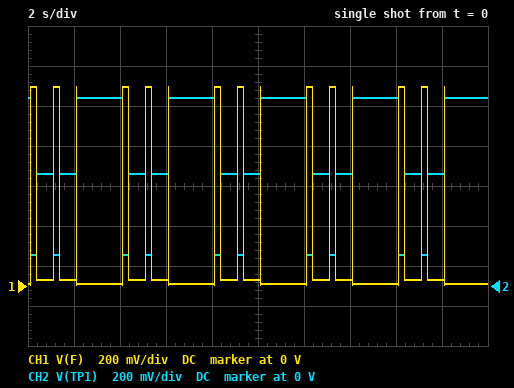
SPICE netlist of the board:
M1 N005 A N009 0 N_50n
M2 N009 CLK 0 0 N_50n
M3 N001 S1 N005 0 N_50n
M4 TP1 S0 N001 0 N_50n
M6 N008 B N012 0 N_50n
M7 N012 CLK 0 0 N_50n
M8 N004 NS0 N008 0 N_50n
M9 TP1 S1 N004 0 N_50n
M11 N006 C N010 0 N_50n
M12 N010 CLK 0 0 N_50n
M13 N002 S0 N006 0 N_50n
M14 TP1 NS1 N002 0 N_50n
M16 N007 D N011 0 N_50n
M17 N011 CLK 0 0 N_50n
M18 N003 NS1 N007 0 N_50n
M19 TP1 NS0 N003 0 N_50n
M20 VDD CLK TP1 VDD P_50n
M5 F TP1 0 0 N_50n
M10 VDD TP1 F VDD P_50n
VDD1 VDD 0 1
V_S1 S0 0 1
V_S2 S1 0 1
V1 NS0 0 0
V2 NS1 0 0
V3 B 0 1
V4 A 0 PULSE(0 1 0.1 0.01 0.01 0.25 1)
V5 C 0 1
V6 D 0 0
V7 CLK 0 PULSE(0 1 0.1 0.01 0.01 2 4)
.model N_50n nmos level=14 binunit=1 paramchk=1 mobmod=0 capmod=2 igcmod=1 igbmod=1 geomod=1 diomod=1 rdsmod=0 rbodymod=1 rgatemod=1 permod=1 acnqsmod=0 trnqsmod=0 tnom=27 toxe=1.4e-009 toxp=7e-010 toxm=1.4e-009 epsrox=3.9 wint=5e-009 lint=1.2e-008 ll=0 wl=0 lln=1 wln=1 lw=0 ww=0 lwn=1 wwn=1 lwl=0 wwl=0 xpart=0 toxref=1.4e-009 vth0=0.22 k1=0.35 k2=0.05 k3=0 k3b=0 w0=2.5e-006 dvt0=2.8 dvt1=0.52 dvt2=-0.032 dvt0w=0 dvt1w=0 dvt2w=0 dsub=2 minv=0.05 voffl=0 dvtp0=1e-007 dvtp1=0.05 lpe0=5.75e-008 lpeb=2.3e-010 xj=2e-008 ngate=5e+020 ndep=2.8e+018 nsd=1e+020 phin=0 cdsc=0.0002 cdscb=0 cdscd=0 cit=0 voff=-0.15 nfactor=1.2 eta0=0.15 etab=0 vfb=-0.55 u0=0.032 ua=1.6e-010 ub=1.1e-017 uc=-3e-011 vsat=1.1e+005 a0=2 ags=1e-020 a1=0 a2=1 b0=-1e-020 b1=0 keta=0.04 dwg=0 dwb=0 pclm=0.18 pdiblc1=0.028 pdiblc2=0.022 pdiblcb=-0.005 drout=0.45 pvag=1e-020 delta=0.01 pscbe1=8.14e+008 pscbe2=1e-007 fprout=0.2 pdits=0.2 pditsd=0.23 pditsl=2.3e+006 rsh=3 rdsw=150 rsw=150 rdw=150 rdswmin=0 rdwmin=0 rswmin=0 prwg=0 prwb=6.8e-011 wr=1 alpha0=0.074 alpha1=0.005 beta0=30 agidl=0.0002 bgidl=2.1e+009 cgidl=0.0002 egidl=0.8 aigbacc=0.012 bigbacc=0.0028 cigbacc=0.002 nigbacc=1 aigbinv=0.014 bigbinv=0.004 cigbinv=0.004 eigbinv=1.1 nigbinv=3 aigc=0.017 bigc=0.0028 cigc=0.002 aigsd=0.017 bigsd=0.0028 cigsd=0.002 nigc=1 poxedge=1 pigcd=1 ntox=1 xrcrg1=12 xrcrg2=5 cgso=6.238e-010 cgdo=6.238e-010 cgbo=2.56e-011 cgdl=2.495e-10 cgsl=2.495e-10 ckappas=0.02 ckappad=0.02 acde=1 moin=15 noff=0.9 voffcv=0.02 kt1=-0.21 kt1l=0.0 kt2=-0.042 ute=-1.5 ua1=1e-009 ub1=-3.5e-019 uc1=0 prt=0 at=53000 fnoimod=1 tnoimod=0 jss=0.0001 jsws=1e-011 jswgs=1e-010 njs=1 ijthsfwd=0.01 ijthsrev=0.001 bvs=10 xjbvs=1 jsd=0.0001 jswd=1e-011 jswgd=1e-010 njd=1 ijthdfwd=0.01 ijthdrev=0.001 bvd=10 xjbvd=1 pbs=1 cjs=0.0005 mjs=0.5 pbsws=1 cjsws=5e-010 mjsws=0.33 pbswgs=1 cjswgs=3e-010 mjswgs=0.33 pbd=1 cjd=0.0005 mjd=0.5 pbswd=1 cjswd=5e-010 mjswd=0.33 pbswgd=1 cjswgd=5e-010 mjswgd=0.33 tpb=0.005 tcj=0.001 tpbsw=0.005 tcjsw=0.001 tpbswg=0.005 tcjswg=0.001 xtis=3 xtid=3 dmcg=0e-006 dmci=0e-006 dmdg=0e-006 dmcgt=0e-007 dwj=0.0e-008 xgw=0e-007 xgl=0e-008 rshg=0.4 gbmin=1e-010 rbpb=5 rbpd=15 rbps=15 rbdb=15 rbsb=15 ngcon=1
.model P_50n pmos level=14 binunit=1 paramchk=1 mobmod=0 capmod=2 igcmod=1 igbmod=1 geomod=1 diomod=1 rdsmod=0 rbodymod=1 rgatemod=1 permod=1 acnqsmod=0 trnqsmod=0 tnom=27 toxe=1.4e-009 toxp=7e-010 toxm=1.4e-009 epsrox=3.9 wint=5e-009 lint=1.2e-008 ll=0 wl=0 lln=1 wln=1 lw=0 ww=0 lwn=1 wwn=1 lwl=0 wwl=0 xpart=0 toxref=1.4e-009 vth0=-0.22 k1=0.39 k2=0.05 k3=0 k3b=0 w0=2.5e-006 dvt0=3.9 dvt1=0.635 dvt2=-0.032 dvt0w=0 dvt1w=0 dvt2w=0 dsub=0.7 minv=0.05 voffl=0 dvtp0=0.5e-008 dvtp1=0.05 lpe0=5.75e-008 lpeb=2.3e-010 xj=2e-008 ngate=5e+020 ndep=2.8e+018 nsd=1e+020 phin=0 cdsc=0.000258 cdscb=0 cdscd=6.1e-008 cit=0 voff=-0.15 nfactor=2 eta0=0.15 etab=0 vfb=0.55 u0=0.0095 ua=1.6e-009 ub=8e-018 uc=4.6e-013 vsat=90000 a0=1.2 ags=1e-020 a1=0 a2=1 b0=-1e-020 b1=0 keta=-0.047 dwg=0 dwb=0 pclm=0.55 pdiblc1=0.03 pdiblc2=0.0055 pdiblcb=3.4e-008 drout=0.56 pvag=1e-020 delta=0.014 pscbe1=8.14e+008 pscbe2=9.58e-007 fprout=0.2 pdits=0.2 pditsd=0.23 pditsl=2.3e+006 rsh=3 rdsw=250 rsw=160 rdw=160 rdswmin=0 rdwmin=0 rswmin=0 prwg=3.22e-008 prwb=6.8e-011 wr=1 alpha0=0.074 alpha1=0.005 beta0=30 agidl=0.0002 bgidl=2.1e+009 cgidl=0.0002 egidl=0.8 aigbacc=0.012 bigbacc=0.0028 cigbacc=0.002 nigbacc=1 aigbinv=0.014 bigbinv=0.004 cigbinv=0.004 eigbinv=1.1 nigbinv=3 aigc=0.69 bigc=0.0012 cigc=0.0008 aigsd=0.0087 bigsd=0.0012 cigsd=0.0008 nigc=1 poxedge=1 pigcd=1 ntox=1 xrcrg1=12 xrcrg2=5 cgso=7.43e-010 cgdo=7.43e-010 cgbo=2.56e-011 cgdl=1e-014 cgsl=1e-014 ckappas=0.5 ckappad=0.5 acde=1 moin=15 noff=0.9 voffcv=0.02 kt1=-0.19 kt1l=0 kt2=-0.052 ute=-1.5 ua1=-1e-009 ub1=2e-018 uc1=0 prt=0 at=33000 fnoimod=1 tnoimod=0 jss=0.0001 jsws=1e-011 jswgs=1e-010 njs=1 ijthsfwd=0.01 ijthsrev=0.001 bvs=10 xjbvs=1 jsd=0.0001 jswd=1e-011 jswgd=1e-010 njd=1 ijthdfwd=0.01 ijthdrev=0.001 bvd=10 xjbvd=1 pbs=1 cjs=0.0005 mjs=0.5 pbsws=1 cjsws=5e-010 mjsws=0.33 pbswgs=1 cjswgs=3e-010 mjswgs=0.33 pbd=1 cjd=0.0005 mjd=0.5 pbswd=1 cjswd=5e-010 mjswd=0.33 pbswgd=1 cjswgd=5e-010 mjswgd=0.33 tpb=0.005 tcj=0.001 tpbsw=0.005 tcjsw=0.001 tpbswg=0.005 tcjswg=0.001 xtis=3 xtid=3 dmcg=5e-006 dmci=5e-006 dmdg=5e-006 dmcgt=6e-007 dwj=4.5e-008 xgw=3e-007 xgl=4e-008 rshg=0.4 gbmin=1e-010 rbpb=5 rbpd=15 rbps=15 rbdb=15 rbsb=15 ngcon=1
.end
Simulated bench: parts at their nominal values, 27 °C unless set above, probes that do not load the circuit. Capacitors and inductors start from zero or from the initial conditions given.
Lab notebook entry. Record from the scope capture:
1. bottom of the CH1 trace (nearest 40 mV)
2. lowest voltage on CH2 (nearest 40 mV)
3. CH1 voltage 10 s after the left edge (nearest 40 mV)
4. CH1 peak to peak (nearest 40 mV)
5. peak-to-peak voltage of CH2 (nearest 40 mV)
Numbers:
0 V
160 mV
40 mV
1.00 V
800 mV
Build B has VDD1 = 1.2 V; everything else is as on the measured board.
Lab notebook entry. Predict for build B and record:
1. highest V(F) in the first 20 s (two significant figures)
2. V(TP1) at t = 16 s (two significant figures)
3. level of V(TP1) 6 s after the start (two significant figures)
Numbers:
1.2 V
1.1 V
600 mV
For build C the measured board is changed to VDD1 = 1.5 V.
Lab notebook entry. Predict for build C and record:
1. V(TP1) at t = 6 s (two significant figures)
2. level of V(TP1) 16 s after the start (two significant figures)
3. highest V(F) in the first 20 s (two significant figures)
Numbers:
1.0 V
1.2 V
1.3 V
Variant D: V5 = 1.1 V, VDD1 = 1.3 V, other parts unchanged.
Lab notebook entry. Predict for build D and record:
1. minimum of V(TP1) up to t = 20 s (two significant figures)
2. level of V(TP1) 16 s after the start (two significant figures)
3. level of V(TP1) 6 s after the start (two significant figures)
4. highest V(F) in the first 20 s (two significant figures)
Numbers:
240 mV
1.1 V
750 mV
1.3 V
